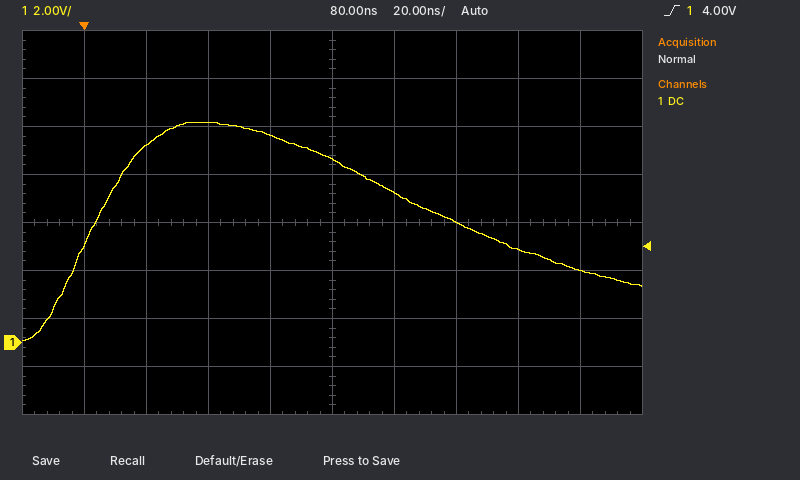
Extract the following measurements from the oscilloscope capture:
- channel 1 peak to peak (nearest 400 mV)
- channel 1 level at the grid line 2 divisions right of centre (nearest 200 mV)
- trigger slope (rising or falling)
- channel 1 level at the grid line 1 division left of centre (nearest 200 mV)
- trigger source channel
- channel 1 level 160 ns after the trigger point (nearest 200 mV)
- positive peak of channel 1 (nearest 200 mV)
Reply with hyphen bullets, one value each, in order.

- 9.2 V
- 5.0 V
- rising
- 8.6 V
- channel 1
- 3.0 V
- 9.2 V
